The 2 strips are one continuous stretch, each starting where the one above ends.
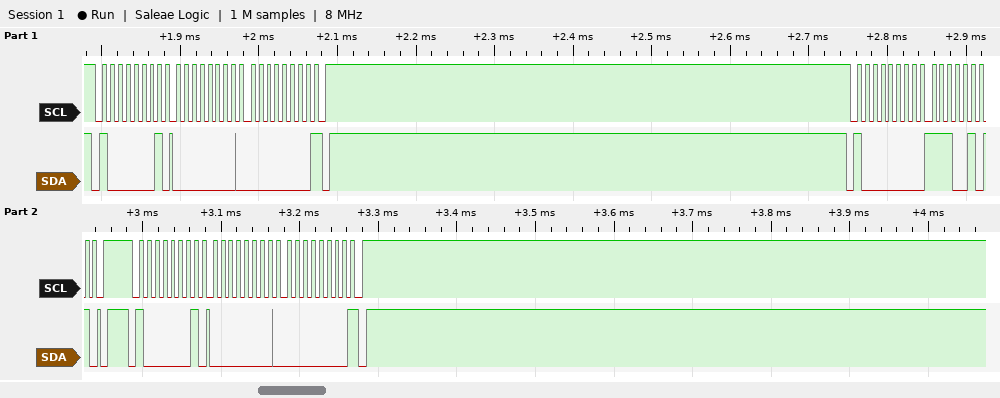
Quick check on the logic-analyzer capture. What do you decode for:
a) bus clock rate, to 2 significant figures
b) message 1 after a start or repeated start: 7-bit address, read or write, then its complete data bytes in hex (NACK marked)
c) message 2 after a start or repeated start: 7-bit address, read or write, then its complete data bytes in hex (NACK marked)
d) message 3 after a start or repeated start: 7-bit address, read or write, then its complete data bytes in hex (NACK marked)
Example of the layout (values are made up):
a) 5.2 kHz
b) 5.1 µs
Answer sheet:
a) 100 kHz
b) 0x40 read: 00 00 NACK
c) 0x40 write: E5
d) 0x40 read: 00 00 NACK
